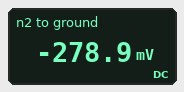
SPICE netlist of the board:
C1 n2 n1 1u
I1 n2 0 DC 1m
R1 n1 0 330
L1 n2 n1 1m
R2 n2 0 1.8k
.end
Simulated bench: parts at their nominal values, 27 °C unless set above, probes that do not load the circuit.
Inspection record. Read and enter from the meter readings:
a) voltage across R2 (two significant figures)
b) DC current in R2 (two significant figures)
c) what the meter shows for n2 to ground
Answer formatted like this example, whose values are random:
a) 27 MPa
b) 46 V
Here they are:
a) 280 mV
b) 150 µA
c) -278.9 mV
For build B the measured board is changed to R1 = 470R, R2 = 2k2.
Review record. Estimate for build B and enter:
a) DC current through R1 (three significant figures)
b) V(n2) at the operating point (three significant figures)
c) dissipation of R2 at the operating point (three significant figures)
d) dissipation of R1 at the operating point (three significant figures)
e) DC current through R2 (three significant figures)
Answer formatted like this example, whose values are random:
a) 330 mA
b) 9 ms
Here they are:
a) 824 µA
b) -387 mV
c) 68.2 µW
d) 319 µW
e) 176 µA
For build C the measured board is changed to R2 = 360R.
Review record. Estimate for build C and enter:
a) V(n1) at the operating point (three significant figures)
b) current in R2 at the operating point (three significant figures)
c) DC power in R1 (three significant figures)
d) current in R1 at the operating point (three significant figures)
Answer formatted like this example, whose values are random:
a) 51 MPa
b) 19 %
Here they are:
a) -172 mV
b) 478 µA
c) 89.8 µW
d) 522 µA
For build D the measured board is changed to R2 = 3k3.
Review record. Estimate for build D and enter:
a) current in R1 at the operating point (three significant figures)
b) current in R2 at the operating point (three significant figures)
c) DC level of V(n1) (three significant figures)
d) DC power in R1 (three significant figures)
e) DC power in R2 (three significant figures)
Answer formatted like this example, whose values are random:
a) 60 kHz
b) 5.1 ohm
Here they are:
a) 909 µA
b) 90.9 µA
c) -300 mV
d) 273 µW
e) 27.3 µW
